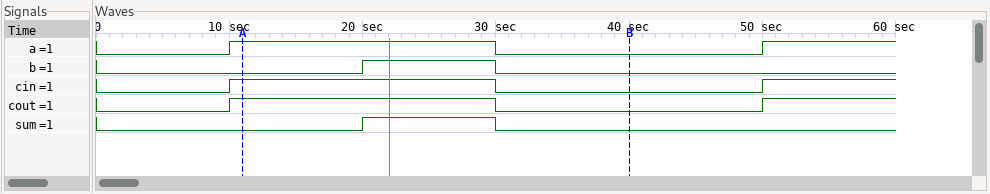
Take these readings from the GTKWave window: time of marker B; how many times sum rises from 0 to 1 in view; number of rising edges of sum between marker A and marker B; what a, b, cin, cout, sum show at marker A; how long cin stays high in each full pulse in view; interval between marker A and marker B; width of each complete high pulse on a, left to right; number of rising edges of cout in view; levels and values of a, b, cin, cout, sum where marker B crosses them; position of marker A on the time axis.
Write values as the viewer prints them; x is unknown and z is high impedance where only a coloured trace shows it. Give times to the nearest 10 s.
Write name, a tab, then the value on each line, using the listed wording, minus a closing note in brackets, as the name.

time of marker B	40 s
how many times sum rises from 0 to 1 in view	1
number of rising edges of sum between marker A and marker B	1
what a, b, cin, cout, sum show at marker A	a=1, b=0, cin=1, cout=1, sum=0
how long cin stays high in each full pulse in view	20 s
interval between marker A and marker B	30 s
width of each complete high pulse on a, left to right	20 s
number of rising edges of cout in view	2
levels and values of a, b, cin, cout, sum where marker B crosses them	a=0, b=0, cin=0, cout=0, sum=0
position of marker A on the time axis	10 s
